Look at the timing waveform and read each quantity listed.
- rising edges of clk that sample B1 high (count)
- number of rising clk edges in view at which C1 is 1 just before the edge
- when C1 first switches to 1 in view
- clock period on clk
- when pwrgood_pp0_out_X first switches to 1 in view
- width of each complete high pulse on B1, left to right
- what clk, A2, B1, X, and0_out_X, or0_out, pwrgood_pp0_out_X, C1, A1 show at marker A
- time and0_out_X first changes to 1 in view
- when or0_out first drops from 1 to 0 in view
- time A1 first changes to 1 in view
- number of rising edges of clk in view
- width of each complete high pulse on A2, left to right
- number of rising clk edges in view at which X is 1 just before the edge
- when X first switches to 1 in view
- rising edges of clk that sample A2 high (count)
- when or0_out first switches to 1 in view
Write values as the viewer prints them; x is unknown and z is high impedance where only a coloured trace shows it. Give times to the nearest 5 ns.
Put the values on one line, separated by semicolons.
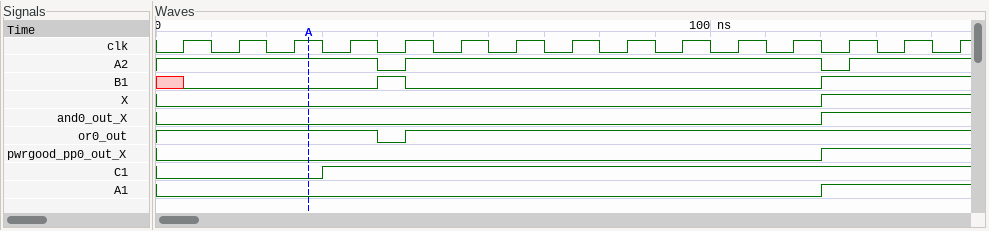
4; 12; 30 ns; 10 ns; 120 ns; 5 ns; clk=1, A2=1, B1=0, X=0, and0_out_X=0, or0_out=1, pwrgood_pp0_out_X=0, C1=0, A1=0; 120 ns; 40 ns; 120 ns; 15; 75 ns; 3; 120 ns; 13; 45 ns
